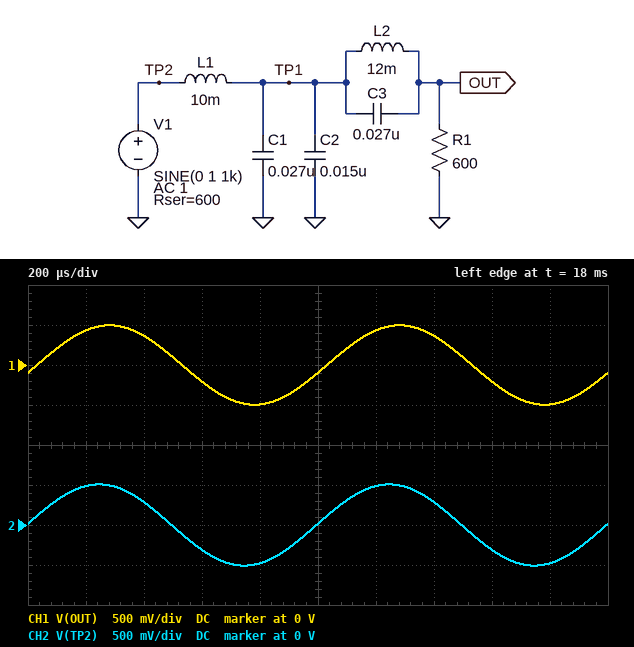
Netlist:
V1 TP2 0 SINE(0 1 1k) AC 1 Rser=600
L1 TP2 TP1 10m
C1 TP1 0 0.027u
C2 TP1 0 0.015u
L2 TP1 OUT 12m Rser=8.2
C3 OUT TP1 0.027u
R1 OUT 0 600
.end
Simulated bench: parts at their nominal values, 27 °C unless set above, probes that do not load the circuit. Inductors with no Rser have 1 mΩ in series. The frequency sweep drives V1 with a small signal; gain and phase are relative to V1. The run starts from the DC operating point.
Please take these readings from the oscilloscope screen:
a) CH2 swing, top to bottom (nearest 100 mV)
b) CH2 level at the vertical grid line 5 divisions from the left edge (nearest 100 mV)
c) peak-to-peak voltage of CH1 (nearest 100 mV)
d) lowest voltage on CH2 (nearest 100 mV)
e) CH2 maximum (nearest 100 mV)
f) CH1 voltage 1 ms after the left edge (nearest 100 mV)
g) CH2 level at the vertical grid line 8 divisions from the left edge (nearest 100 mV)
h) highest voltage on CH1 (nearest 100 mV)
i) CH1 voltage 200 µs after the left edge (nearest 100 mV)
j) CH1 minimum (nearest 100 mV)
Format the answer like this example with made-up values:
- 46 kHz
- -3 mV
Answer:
- 1.0 V
- 0 V
- 1.0 V
- -500 mV
- 500 mV
- -100 mV
- -300 mV
- 500 mV
- 400 mV
- -500 mV
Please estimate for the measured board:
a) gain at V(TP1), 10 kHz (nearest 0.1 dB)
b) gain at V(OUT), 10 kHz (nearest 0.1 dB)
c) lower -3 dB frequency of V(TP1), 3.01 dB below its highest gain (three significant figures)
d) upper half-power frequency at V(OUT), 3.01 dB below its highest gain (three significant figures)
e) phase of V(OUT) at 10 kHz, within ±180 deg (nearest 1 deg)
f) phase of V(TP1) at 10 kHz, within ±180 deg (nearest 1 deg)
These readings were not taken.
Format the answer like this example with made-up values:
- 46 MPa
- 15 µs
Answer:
- -6.1 dB
- -19.5 dB
- 5.03 kHz
- 7.06 kHz
- -39 deg
- -114 deg
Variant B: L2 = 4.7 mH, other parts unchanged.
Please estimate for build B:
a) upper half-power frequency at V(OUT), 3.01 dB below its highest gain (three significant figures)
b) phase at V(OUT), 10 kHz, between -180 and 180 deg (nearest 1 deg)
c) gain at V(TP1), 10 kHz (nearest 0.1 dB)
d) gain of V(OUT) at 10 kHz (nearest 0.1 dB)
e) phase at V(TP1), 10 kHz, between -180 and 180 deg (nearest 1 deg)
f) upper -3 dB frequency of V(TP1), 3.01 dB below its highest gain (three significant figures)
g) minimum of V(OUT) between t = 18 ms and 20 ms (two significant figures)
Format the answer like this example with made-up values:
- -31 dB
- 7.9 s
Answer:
- 10.8 kHz
- -121 deg
- -4.5 dB
- -7.7 dB
- -78 deg
- 12.9 kHz
- -500 mV
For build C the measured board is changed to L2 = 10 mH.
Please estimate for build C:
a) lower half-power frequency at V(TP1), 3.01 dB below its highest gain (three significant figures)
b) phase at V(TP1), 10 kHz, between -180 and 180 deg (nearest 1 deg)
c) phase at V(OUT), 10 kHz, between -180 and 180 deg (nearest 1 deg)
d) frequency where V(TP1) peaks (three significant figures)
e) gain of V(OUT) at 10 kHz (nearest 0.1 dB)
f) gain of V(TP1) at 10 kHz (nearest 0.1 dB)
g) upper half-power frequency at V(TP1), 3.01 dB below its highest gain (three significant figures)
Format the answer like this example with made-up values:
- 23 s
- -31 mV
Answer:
- 5.29 kHz
- -113 deg
- -38 deg
- 7.86 kHz
- -29.1 dB
- -5.1 dB
- 9.56 kHz
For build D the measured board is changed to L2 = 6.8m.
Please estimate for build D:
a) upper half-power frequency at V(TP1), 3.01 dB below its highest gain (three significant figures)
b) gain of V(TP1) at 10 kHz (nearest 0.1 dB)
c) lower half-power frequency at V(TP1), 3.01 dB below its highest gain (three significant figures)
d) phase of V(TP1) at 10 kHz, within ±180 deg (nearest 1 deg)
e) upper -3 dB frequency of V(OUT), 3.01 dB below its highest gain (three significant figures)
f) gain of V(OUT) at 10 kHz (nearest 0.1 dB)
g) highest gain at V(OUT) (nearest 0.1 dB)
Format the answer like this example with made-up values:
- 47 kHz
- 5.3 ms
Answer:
- 11.1 kHz
- -3.1 dB
- 4.27 kHz
- -97 deg
- 9.37 kHz
- -12.1 dB
- -6.1 dB
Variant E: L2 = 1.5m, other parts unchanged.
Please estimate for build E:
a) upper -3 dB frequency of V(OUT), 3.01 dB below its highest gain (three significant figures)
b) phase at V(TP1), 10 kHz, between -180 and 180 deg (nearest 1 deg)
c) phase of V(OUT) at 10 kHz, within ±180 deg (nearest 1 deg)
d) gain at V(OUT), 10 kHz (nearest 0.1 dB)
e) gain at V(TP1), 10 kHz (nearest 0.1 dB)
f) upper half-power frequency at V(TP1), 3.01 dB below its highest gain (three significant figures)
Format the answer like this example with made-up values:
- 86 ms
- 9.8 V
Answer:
- 11.4 kHz
- -79 deg
- -89 deg
- -8.1 dB
- -7.8 dB
- 11.8 kHz
